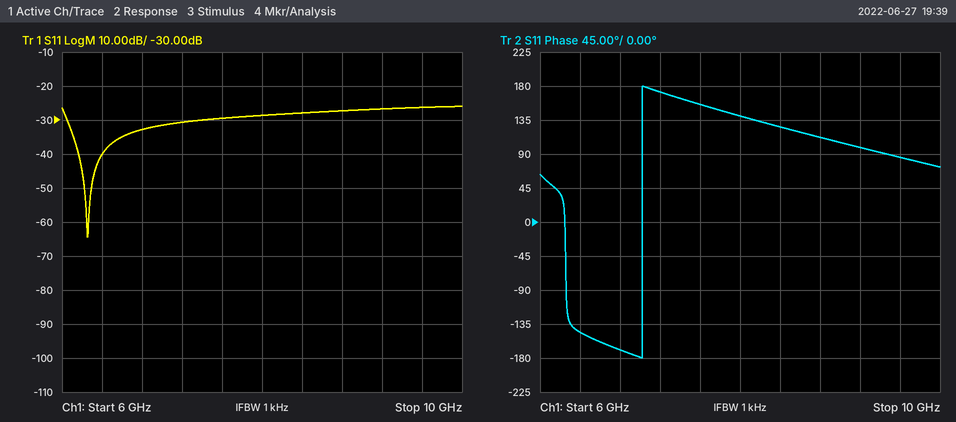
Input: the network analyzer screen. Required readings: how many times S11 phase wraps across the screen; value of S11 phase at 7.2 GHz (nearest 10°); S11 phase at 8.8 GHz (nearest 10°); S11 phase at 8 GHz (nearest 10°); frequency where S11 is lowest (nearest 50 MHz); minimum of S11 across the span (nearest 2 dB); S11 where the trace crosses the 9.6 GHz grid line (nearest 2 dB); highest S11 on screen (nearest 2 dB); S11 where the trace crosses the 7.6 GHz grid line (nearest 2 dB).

1
170°
110°
140°
6.25 GHz
-64 dB
-26 dB
-26 dB
-30 dB
